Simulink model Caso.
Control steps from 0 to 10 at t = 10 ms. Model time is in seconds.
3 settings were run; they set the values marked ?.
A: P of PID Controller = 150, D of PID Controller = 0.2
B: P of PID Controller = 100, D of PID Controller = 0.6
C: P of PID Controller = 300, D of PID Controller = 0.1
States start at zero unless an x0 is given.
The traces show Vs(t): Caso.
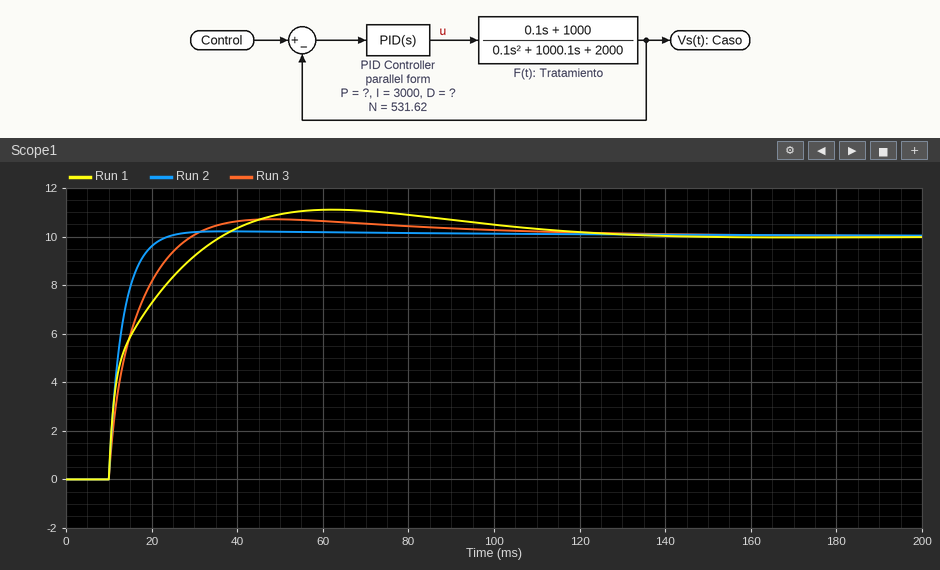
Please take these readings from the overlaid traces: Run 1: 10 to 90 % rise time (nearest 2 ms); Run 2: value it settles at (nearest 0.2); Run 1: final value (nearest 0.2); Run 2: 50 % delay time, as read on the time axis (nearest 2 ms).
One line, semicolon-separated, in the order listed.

18 ms; 10.0; 10.0; 12 ms
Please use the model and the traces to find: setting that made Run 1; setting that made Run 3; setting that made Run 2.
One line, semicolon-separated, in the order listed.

B; A; C
